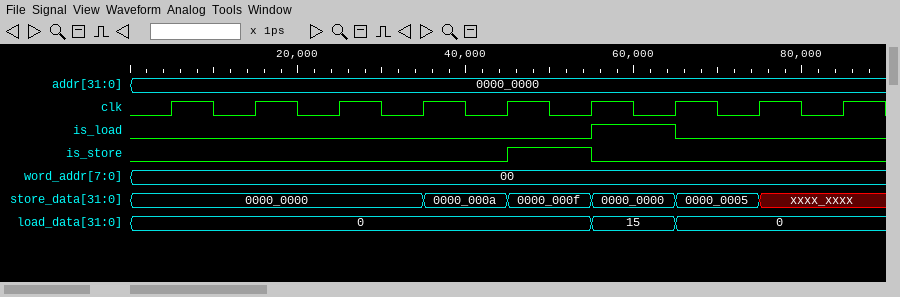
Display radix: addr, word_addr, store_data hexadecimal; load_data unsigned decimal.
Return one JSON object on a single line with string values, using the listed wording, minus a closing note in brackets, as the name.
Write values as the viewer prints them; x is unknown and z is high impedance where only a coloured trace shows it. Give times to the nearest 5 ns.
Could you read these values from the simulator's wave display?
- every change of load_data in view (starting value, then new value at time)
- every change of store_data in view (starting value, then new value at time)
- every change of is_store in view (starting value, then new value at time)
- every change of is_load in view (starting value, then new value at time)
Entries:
{"every change of load_data in view": "0, 15 at 55 ns, 0 at 65 ns", "every change of store_data in view": "0000_0000, 0000_000a at 35 ns, 0000_000f at 45 ns, 0000_0000 at 55 ns, 0000_0005 at 65 ns, xxxx_xxxx at 75 ns", "every change of is_store in view": "0, 1 at 45 ns, 0 at 55 ns", "every change of is_load in view": "0, 1 at 55 ns, 0 at 65 ns"}
